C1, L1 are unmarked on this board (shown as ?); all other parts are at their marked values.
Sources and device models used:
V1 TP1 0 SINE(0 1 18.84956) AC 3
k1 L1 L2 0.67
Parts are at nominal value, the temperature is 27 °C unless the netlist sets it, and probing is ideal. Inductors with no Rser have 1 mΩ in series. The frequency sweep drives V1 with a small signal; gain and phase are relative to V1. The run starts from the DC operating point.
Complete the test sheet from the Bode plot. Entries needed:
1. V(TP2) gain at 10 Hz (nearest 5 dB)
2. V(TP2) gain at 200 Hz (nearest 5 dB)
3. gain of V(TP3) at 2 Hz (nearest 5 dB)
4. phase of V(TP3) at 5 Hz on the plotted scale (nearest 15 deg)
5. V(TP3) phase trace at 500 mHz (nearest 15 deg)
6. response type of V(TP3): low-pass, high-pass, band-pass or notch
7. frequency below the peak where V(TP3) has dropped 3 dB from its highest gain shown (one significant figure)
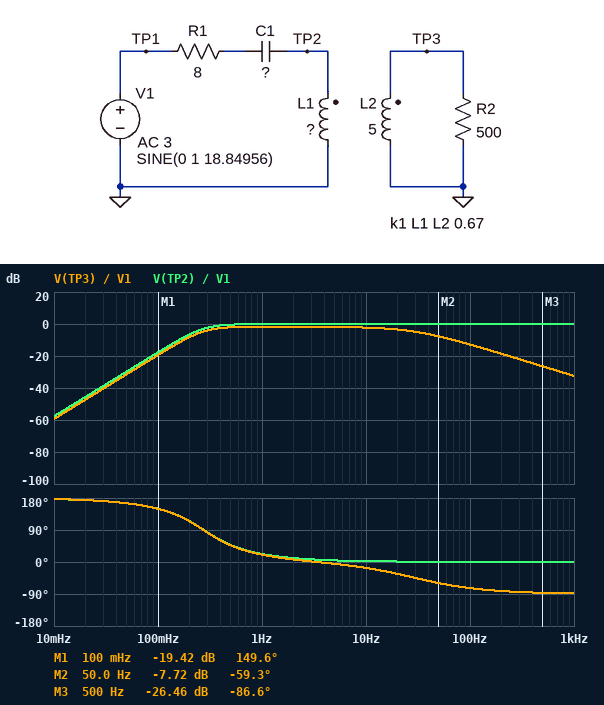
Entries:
0 dB
0 dB
0 dB
0 deg
45 deg
band-pass
300 mHz
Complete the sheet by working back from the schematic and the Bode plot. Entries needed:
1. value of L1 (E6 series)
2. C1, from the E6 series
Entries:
3.3 H
100 mF
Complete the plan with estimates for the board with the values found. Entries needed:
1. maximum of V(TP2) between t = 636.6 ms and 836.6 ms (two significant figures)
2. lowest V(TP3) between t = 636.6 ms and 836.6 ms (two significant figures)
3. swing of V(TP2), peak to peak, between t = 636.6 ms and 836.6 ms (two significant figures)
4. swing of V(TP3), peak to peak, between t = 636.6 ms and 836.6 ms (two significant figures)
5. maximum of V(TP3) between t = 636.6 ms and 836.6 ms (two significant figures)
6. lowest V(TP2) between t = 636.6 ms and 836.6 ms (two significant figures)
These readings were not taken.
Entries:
990 mV
-690 mV
2.0 V
1.4 V
680 mV
-1.0 V
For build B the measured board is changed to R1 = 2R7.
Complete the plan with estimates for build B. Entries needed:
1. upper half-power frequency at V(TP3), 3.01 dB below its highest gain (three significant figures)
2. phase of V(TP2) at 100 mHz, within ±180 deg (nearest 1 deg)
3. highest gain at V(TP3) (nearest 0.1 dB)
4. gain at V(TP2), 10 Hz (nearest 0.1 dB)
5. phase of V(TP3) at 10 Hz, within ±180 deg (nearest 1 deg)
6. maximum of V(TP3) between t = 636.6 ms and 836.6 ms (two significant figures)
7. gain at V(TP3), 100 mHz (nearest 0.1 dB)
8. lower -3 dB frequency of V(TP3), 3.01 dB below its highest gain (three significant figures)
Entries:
425 mHz
169 deg
5.0 dB
0 dB
-18 deg
680 mV
-18.3 dB
238 mHz
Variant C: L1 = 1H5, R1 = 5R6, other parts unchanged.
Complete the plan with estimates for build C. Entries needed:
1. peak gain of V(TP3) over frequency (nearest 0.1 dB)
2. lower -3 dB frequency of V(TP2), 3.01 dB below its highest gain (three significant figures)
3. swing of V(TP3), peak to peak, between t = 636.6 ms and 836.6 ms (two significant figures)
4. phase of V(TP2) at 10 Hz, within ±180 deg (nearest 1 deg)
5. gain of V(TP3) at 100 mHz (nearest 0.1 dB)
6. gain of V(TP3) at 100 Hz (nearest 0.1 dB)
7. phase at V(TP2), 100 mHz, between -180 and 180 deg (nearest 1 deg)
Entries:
1.6 dB
424 mHz
2.0 V
4 deg
-22.8 dB
-9.4 dB
159 deg
